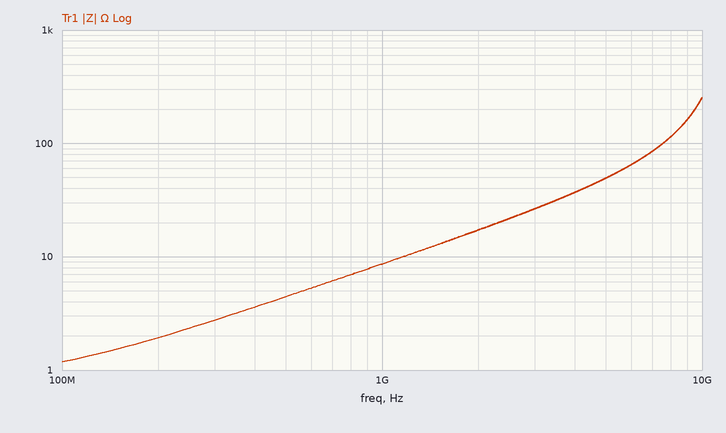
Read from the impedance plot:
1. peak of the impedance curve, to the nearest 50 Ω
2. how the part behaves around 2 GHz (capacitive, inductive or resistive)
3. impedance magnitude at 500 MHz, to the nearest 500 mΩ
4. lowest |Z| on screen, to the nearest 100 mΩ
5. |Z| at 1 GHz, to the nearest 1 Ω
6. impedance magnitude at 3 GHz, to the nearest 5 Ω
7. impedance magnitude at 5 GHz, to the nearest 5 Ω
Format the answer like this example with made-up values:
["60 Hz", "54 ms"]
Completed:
["250 Ω", "inductive", "4.5 Ω", "1.2 Ω", "9 Ω", "25 Ω", "50 Ω"]
